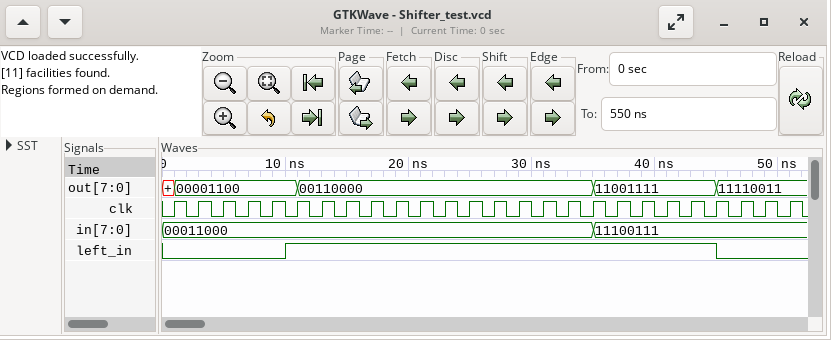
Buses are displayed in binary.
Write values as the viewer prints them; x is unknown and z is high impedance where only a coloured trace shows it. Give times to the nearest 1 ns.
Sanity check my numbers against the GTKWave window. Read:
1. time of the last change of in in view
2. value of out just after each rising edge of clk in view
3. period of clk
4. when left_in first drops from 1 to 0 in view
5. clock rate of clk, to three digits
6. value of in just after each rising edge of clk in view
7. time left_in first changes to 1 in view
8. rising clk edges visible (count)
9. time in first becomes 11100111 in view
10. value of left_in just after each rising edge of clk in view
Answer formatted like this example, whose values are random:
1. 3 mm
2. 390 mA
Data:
1. 35 ns
2. 00001100, 00001100, 00001100, 00001100, 00001100, 00110000, 00110000, 00110000, 00110000, 00110000, 00110000, 00110000, 00110000, 00110000, 00110000, 00110000, 00110000, 11001111, 11001111, 11001111, 11001111, 11001111, 11110011, 11110011, 11110011, 11110011
3. 2 ns
4. 45 ns
5. 500 MHz
6. 00011000, 00011000, 00011000, 00011000, 00011000, 00011000, 00011000, 00011000, 00011000, 00011000, 00011000, 00011000, 00011000, 00011000, 00011000, 00011000, 00011000, 11100111, 11100111, 11100111, 11100111, 11100111, 11100111, 11100111, 11100111, 11100111
7. 10 ns
8. 26
9. 35 ns
10. 0 0 0 0 0 1 1 1 1 1 1 1 1 1 1 1 1 1 1 1 1 1 0 0 0 0
